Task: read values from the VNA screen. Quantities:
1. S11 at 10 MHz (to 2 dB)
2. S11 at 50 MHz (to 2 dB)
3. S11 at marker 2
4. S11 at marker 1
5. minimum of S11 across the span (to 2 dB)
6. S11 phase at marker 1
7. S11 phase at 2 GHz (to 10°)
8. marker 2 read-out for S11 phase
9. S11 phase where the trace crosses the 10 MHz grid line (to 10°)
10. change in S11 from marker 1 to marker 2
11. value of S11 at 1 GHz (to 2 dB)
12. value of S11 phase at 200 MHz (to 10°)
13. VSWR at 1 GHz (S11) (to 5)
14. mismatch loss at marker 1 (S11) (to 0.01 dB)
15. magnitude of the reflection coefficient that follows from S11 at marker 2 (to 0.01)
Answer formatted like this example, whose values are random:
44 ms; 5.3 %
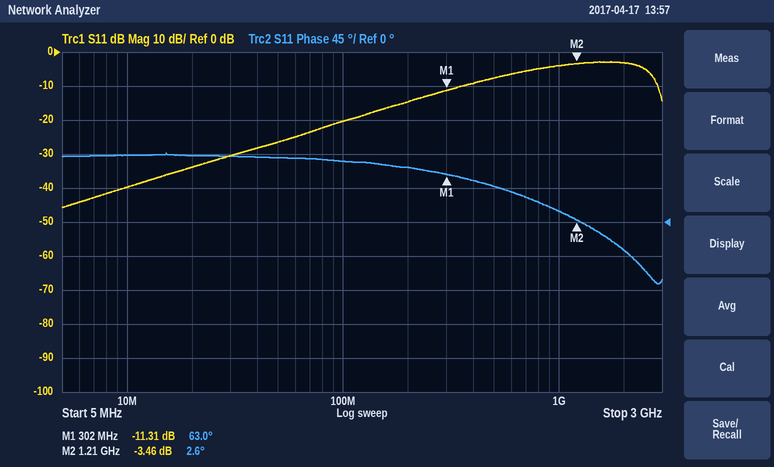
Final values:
-40 dB; -26 dB; -3.46 dB; -11.31 dB; -46 dB; 63.0°; -40°; 2.6°; 90°; 7.85 dB; -4 dB; 70°; 5; 0.33 dB; 0.67
